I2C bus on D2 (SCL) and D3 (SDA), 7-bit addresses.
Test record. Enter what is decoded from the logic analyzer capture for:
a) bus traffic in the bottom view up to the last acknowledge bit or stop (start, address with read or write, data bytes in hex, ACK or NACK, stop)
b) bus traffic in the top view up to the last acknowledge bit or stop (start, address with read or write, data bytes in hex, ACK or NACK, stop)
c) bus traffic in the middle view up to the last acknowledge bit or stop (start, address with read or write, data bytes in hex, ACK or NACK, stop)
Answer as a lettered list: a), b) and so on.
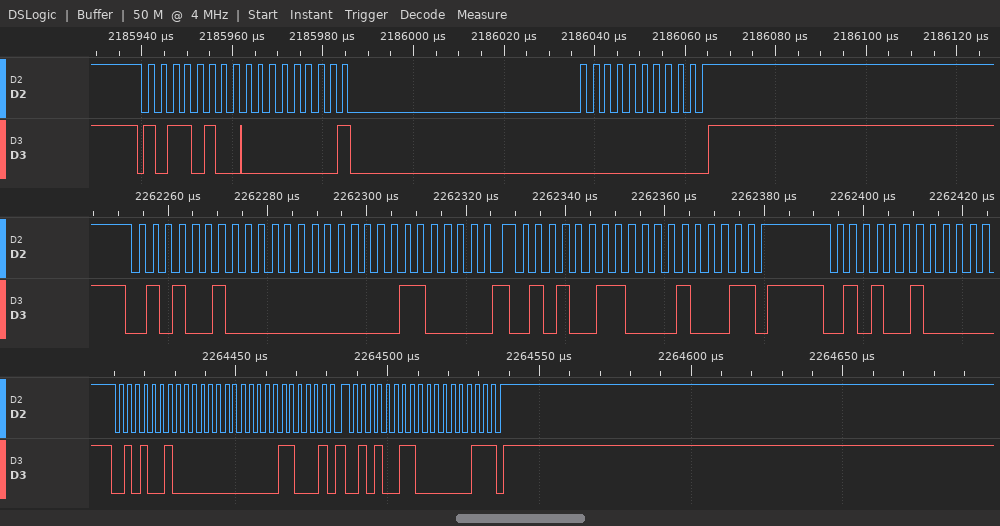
a) start, address 29 write ACK, 00 ACK, 31 ACK, repeated start, address 29 read ACK, 03 NACK, stop
b) start, address 5A write ACK, 01 ACK, 00 ACK, stop
c) start, address 29 write ACK, 00 ACK, 30 ACK, repeated start, address 29 read ACK, 11 NACK, stop, start, address 29 write ACK
